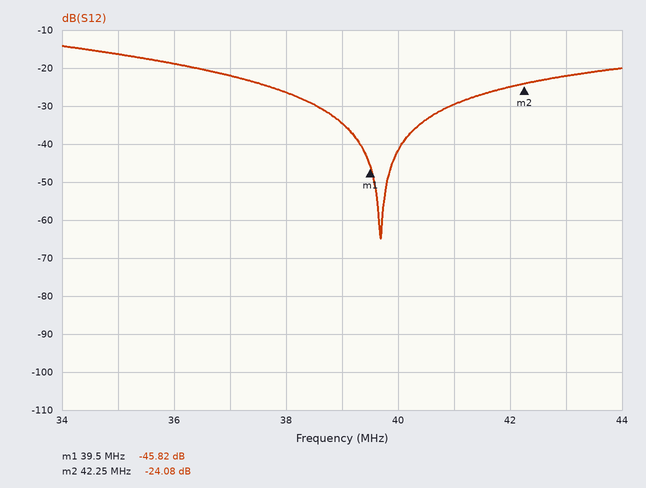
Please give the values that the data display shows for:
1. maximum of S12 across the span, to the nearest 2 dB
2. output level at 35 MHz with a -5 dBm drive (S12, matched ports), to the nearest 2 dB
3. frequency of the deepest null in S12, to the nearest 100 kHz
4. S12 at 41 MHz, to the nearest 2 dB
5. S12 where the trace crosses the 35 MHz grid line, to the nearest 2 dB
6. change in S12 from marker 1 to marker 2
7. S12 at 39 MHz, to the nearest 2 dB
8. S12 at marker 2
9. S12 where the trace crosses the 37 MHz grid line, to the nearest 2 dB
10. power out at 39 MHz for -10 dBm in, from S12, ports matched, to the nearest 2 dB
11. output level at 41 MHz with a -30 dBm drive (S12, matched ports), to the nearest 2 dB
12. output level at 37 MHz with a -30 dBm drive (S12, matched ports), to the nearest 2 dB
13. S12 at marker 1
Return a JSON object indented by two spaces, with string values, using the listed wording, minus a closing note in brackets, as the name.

{
  "maximum of S12 across the span, to the nearest 2 dB": "-14 dB",
  "output level at 35 MHz with a -5 dBm drive (S12, matched ports), to the nearest 2 dB": "-22 dBm",
  "frequency of the deepest null in S12, to the nearest 100 kHz": "39.7 MHz",
  "S12 at 41 MHz, to the nearest 2 dB": "-30 dB",
  "S12 where the trace crosses the 35 MHz grid line, to the nearest 2 dB": "-16 dB",
  "change in S12 from marker 1 to marker 2": "21.74 dB",
  "S12 at 39 MHz, to the nearest 2 dB": "-34 dB",
  "S12 at marker 2": "-24.08 dB",
  "S12 where the trace crosses the 37 MHz grid line, to the nearest 2 dB": "-22 dB",
  "power out at 39 MHz for -10 dBm in, from S12, ports matched, to the nearest 2 dB": "-44 dBm",
  "output level at 41 MHz with a -30 dBm drive (S12, matched ports), to the nearest 2 dB": "-60 dBm",
  "output level at 37 MHz with a -30 dBm drive (S12, matched ports), to the nearest 2 dB": "-52 dBm",
  "S12 at marker 1": "-45.82 dB"
}
